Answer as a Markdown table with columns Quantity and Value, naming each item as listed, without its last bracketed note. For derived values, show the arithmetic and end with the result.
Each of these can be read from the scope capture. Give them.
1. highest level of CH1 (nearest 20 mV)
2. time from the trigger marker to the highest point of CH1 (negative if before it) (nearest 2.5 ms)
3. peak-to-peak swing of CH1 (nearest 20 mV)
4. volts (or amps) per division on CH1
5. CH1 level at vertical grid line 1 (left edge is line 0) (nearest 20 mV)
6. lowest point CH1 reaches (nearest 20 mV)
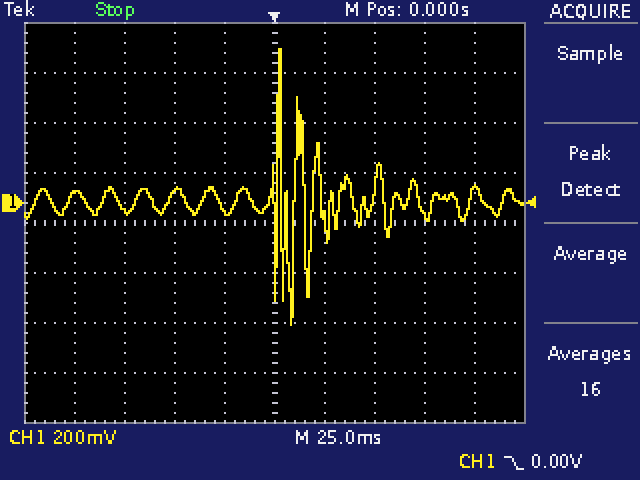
| Quantity | Value |
|---|---|
| highest level of CH1 | 620 mV |
| time from the trigger marker to the highest point of CH1 (negative if before it) | +2.5 ms |
| peak-to-peak swing of CH1 | 620 mV − (-480 mV) = 1.10 V |
| volts (or amps) per division on CH1 | 200 mV |
| CH1 level at vertical grid line 1 (left edge is line 0) | 40 mV |
| lowest point CH1 reaches | -480 mV |
